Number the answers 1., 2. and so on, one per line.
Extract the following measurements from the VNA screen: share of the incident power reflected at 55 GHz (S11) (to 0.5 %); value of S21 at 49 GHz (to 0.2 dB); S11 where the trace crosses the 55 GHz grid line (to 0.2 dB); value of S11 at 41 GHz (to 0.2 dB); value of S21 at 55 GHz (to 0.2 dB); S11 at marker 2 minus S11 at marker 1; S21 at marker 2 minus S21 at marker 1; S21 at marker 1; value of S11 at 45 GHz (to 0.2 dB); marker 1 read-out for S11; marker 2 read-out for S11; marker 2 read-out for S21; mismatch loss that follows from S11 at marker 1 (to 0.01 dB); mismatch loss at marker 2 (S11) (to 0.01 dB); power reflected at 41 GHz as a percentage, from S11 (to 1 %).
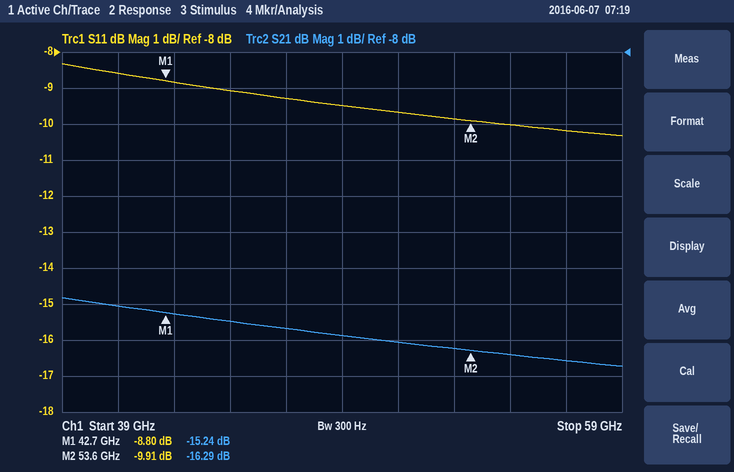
1. 10.0 %
2. -15.8 dB
3. -10.0 dB
4. -8.6 dB
5. -16.4 dB
6. -1.11 dB
7. -1.05 dB
8. -15.24 dB
9. -9.0 dB
10. -8.80 dB
11. -9.91 dB
12. -16.29 dB
13. 0.61 dB
14. 0.47 dB
15. 14 %
